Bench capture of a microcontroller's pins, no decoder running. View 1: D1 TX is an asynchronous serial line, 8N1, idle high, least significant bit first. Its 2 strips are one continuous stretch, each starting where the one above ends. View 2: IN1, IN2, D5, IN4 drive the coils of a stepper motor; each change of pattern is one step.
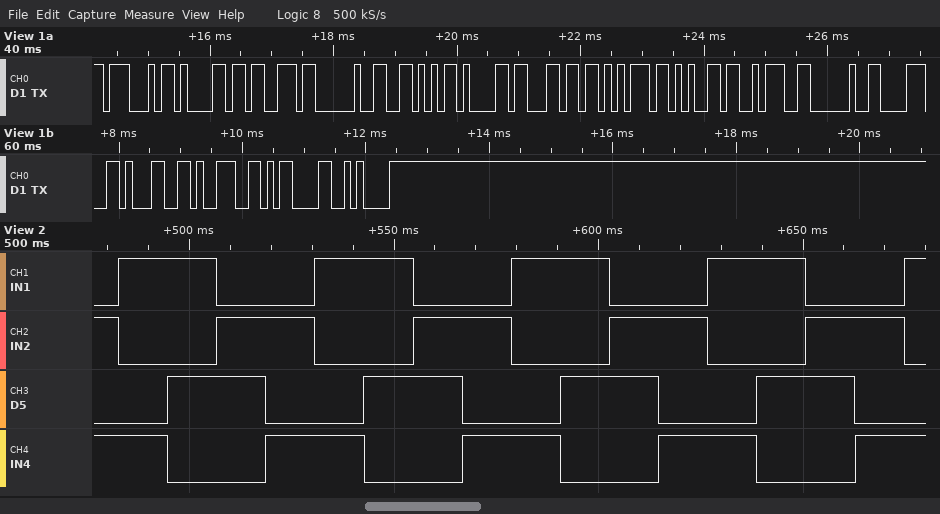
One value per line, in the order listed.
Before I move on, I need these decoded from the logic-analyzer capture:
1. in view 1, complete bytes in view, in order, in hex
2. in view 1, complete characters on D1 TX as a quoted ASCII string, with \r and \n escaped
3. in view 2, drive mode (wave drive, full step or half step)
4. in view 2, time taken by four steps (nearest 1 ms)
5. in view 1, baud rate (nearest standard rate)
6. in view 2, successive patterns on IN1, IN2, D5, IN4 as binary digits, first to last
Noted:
47 61 73 20 56 61 6C 75 65 3A 20 38 31 39 0D 0A
"Gas Value: 819\r\n"
full step
48 ms
9600 baud
0101 1001 1010 0110 0101 1001 1010 0110 0101 1001 1010 0110 0101 1001 1010 0110 0101 1001
